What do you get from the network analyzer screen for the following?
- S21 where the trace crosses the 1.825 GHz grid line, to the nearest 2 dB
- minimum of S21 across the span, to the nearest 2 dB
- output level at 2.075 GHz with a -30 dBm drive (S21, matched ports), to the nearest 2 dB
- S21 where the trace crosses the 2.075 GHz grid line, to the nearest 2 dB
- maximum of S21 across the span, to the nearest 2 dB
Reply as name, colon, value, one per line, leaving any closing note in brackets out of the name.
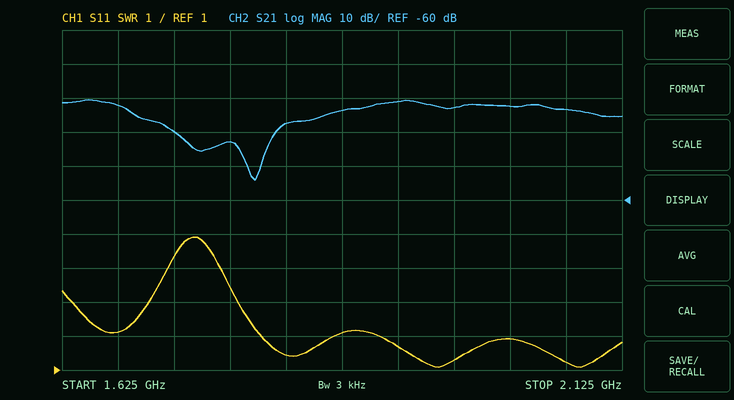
S21 where the trace crosses the 1.825 GHz grid line, to the nearest 2 dB: -38 dB
minimum of S21 across the span, to the nearest 2 dB: -54 dB
output level at 2.075 GHz with a -30 dBm drive (S21, matched ports), to the nearest 2 dB: -64 dBm
S21 where the trace crosses the 2.075 GHz grid line, to the nearest 2 dB: -34 dB
maximum of S21 across the span, to the nearest 2 dB: -30 dB
